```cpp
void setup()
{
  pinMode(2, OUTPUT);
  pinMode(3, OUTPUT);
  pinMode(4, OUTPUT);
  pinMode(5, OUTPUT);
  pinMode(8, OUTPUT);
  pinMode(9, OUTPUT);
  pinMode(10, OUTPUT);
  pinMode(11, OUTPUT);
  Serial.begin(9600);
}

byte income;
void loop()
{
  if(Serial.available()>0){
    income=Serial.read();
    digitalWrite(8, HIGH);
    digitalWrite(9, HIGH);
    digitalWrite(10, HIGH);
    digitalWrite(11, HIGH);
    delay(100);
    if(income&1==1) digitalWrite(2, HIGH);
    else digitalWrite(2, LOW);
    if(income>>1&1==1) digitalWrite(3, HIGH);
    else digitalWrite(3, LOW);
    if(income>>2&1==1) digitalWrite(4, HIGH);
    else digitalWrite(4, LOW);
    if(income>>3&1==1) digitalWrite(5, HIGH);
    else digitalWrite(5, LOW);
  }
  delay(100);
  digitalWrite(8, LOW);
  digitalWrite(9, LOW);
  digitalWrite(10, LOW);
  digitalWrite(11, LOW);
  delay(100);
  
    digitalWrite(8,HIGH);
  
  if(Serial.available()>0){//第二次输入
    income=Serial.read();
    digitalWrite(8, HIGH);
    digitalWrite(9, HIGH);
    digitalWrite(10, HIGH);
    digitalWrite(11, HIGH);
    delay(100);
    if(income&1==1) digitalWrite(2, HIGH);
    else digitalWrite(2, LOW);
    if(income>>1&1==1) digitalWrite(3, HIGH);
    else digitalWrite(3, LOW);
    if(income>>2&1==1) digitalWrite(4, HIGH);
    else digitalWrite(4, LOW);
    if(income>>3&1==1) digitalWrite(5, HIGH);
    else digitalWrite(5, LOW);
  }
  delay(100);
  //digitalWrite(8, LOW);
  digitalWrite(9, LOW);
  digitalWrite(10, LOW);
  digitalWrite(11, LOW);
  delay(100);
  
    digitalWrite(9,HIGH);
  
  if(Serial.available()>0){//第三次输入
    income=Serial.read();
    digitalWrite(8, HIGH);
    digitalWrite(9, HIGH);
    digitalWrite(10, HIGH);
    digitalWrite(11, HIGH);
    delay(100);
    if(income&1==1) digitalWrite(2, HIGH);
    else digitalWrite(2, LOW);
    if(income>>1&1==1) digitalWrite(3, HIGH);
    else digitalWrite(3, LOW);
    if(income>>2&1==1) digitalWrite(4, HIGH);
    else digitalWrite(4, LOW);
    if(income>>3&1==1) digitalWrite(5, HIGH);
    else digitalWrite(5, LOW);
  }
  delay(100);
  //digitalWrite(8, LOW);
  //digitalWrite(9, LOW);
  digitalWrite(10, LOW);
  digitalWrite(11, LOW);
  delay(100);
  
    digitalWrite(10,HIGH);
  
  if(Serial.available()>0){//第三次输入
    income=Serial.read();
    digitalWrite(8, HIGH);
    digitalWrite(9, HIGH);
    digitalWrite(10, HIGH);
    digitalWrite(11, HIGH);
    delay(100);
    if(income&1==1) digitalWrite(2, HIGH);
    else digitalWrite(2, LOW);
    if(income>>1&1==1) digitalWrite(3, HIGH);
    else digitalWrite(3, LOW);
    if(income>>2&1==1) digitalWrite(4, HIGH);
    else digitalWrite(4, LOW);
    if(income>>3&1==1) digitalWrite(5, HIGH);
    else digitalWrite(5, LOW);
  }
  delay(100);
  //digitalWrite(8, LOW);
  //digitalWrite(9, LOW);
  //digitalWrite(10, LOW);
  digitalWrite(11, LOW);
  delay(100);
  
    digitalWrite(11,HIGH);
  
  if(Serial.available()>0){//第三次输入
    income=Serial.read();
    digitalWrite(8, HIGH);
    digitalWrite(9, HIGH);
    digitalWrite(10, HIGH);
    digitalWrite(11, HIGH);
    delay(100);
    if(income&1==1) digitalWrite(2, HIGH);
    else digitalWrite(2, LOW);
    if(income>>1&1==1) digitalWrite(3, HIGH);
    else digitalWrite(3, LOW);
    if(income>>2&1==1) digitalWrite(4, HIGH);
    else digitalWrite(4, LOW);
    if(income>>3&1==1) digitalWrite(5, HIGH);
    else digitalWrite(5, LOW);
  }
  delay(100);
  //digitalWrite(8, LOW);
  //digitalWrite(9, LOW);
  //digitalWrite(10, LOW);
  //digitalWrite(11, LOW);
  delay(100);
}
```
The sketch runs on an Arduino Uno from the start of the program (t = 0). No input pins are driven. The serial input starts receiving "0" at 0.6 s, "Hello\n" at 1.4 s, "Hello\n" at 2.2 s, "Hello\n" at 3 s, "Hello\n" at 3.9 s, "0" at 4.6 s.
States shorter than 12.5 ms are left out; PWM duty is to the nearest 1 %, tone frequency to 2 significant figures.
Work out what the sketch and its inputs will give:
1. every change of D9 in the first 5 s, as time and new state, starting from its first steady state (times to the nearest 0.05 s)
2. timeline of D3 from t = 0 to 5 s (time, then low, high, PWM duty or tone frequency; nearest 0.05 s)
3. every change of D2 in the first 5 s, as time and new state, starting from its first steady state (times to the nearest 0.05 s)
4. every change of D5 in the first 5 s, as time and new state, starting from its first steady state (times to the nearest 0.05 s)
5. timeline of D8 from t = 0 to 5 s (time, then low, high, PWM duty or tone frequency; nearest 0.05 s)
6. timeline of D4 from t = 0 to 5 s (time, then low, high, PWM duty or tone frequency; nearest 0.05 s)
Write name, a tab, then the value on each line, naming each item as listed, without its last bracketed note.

every change of D9 in the first 5 s, as time and new state, starting from its first steady state	0 s low; 0.4 s high; 1.2 s low; 1.5 s high; 2.6 s low; 2.7 s high; 2.9 s low; 3 s high; 4.1 s low; 4.2 s high; 4.4 s low; 4.5 s high
timeline of D3 from t = 0 to 5 s	0 s low; 2.8 s high; 3.4 s low; 4.6 s high
every change of D2 in the first 5 s, as time and new state, starting from its first steady state	0 s low; 1.9 s high; 2.2 s low; 2.8 s high; 3.1 s low; 3.7 s high; 4 s low; 4.6 s high; 4.9 s low
every change of D5 in the first 5 s, as time and new state, starting from its first steady state	0 s low; 1.6 s high; 1.9 s low; 2.2 s high; 3.7 s low; 4 s high
timeline of D8 from t = 0 to 5 s	0 s low; 0.2 s high; 1.2 s low; 1.3 s high; 2.6 s low; 2.7 s high; 4.1 s low; 4.2 s high
timeline of D4 from t = 0 to 5 s	0 s low; 1.9 s high; 3.1 s low; 3.7 s high; 4.9 s low
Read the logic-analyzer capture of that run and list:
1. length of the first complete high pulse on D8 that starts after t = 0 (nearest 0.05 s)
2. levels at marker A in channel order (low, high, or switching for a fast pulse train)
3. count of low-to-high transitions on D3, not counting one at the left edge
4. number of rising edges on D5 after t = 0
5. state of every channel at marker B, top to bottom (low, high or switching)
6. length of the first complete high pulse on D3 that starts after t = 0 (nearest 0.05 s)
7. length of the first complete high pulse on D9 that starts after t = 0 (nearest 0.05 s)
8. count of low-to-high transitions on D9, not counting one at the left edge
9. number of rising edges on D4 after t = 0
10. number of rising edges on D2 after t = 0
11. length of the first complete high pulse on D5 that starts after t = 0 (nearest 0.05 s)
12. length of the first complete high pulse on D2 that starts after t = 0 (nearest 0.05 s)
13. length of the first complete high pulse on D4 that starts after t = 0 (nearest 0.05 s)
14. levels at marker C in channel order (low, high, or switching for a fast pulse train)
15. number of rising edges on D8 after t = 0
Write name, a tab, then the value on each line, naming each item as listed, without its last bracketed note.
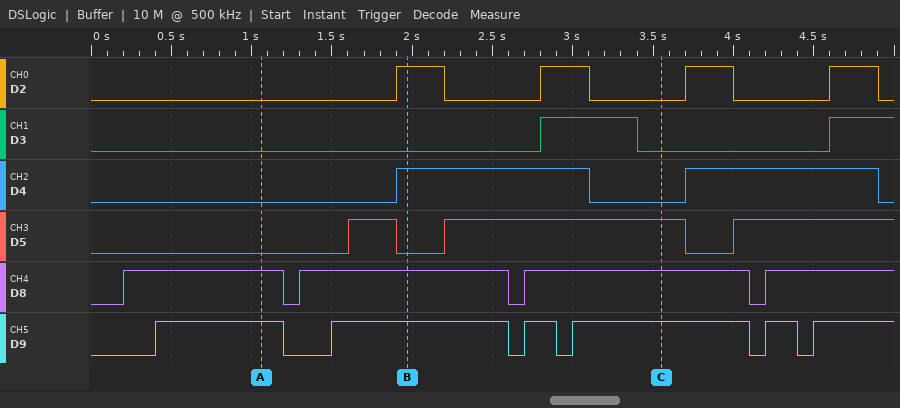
length of the first complete high pulse on D8 that starts after t = 0	1.00 s
levels at marker A in channel order	D2 low, D3 low, D4 low, D5 low, D8 high, D9 high
count of low-to-high transitions on D3, not counting one at the left edge	2
number of rising edges on D5 after t = 0	3
state of every channel at marker B, top to bottom	D2 high, D3 low, D4 high, D5 low, D8 high, D9 high
length of the first complete high pulse on D3 that starts after t = 0	0.60 s
length of the first complete high pulse on D9 that starts after t = 0	0.80 s
count of low-to-high transitions on D9, not counting one at the left edge	6
number of rising edges on D4 after t = 0	2
number of rising edges on D2 after t = 0	4
length of the first complete high pulse on D5 that starts after t = 0	0.30 s
length of the first complete high pulse on D2 that starts after t = 0	0.30 s
length of the first complete high pulse on D4 that starts after t = 0	1.20 s
levels at marker C in channel order	D2 low, D3 low, D4 low, D5 high, D8 high, D9 high
number of rising edges on D8 after t = 0	4
